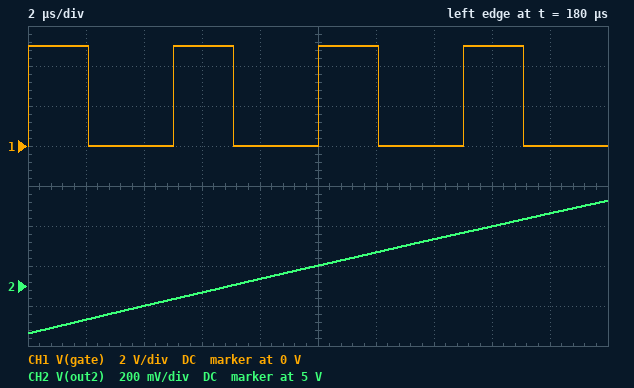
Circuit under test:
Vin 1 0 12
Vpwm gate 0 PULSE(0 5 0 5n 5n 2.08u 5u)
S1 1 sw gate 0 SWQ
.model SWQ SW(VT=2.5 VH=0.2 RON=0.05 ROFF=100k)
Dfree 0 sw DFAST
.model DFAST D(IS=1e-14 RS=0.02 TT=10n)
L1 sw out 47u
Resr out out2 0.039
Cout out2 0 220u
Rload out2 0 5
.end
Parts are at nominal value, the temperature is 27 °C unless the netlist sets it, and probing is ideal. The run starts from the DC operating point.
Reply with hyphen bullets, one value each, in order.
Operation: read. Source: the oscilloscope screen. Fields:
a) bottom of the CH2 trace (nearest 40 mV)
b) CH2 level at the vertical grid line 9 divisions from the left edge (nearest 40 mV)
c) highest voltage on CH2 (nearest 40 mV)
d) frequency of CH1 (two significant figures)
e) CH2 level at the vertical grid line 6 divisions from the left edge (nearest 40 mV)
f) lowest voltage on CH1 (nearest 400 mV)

- 4.76 V
- 5.36 V
- 5.44 V
- 200 kHz
- 5.16 V
- 0 V
